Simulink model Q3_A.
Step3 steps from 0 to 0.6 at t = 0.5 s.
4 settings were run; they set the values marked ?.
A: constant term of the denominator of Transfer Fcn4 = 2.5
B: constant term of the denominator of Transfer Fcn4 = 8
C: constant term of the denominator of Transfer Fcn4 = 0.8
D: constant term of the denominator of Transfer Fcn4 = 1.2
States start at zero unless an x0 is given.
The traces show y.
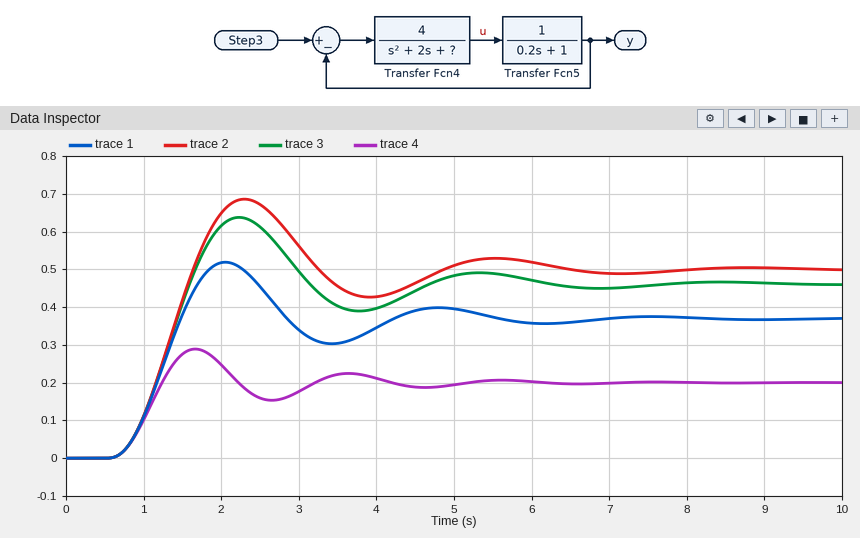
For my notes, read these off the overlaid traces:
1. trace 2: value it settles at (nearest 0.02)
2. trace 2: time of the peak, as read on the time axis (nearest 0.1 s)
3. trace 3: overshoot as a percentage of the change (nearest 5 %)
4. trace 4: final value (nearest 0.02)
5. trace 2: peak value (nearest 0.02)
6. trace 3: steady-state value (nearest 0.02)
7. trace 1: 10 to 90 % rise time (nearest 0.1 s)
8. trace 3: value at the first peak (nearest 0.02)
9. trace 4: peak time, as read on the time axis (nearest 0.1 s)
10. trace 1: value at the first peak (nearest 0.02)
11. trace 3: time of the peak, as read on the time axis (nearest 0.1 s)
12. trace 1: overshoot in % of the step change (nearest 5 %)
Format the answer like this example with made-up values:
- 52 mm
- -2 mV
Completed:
- 0.50
- 2.3 s
- 40 %
- 0.20
- 0.68
- 0.46
- 0.6 s
- 0.64
- 1.7 s
- 0.52
- 2.2 s
- 40 %
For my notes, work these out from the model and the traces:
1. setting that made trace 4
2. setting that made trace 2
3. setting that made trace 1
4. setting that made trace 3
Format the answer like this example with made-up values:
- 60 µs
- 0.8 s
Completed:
- B
- C
- A
- D
